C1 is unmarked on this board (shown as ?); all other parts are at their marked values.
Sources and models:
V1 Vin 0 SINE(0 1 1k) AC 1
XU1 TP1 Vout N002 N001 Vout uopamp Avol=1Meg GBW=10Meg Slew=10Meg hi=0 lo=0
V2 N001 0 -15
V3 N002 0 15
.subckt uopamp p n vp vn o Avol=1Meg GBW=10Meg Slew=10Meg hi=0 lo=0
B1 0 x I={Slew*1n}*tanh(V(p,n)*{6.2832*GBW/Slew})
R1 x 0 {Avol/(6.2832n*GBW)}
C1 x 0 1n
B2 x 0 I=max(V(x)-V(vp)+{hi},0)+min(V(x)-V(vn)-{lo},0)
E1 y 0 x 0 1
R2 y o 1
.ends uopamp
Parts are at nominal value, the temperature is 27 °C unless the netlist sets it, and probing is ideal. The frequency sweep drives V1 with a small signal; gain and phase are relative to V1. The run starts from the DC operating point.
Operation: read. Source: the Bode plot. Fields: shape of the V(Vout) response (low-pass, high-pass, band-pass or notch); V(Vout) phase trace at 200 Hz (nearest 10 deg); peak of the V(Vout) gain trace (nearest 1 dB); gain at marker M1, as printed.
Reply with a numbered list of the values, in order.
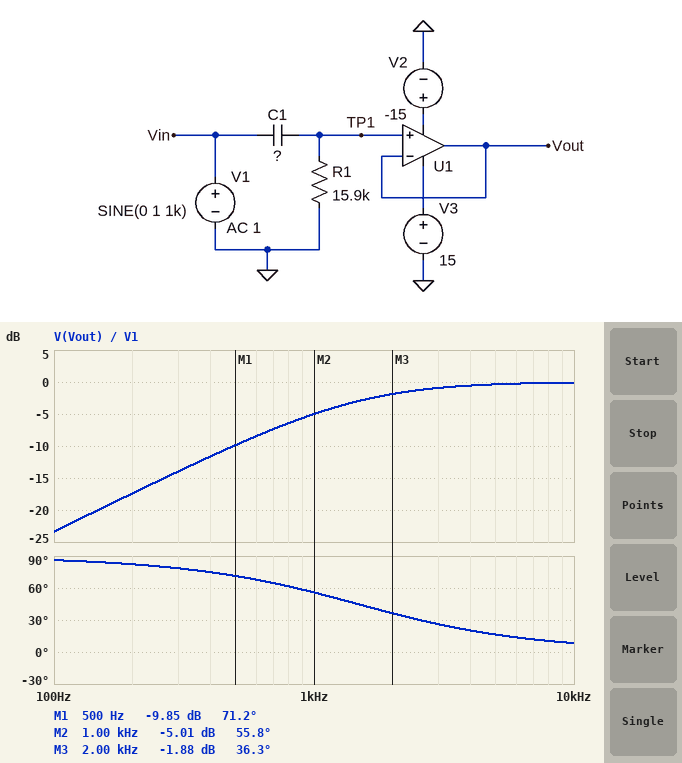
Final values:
1. high-pass
2. 80 deg
3. 0 dB
4. -9.85 dB
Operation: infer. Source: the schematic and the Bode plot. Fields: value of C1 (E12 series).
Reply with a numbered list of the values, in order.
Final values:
1. 6.8 nF
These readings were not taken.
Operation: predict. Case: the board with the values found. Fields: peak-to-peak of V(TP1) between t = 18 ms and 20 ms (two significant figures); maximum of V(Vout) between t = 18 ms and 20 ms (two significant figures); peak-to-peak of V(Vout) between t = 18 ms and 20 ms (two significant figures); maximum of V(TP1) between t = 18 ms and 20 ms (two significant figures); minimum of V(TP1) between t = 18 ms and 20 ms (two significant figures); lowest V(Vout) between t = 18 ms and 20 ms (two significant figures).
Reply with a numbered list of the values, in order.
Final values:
1. 1.1 V
2. 560 mV
3. 1.1 V
4. 560 mV
5. -560 mV
6. -560 mV
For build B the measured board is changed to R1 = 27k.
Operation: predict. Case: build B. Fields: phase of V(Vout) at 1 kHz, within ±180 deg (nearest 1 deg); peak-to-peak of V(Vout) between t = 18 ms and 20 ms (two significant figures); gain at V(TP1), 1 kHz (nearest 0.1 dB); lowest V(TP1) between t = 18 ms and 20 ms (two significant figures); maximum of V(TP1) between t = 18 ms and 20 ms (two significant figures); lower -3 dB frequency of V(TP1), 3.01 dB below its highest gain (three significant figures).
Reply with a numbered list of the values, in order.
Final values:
1. 41 deg
2. 1.5 V
3. -2.4 dB
4. -760 mV
5. 760 mV
6. 867 Hz
